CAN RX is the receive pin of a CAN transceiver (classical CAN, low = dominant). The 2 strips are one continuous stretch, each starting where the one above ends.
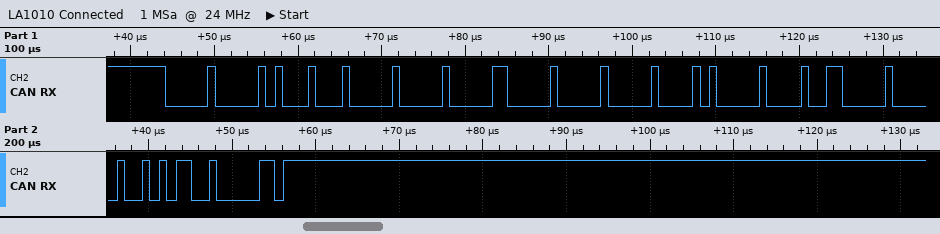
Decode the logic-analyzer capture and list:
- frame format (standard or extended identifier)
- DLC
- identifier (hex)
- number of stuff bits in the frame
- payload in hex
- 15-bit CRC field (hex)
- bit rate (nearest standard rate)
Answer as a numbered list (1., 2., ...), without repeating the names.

1. standard
2. 8
3. 0x001
4. 12
5. 80 00 80 00 0A 00 98 00
6. 0x2B20
7. 1000 kbit/s
